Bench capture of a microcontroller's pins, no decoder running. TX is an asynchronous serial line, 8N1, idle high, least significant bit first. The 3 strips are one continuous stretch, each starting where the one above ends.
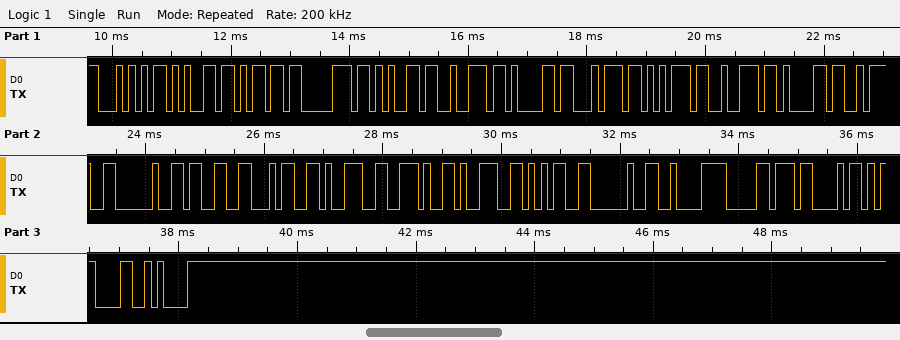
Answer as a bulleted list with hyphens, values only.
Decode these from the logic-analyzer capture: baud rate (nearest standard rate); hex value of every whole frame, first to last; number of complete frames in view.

- 9600 baud
- 0x54 0x65 0x6D 0x70 0x65 0x72 0x61 0x74 0x75 0x72 0x61 0x3A 0x20 0x33 0x34 0x39 0x2E 0x39 0x35 0x20 0xC2 0xB0 0x43 0x0D 0x0A
- 25
